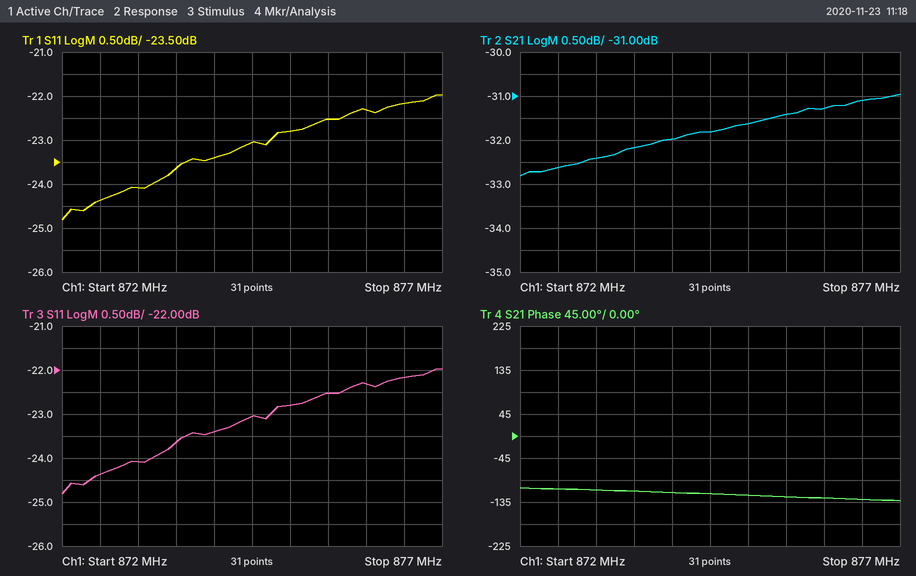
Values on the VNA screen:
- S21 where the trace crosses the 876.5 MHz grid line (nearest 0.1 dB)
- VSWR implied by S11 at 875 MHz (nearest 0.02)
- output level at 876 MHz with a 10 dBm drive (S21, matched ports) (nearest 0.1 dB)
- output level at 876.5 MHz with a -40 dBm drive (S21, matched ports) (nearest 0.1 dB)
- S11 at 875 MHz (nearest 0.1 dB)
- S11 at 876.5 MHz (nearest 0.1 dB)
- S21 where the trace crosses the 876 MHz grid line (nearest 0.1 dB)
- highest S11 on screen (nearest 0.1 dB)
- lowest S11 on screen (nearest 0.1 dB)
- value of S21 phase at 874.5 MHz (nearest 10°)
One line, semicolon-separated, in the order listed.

-31.1 dB; 1.16; -21.3 dBm; -71.1 dBm; -22.8 dB; -22.2 dB; -31.3 dB; -22.0 dB; -24.8 dB; -120°
